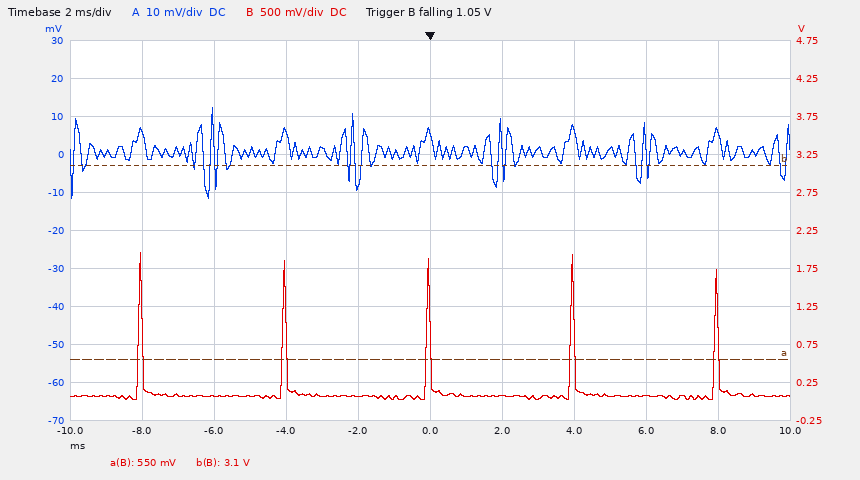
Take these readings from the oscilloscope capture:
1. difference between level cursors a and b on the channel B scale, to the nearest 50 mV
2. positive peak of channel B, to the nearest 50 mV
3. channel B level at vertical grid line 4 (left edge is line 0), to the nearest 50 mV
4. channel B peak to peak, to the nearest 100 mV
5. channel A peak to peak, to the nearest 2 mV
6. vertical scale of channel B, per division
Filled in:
2.55 V
1.95 V
50 mV
1.90 V
24 mV
500 mV
